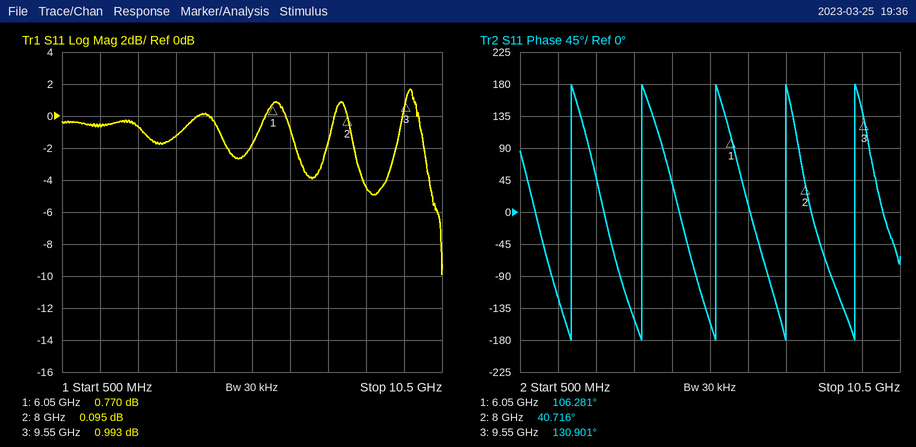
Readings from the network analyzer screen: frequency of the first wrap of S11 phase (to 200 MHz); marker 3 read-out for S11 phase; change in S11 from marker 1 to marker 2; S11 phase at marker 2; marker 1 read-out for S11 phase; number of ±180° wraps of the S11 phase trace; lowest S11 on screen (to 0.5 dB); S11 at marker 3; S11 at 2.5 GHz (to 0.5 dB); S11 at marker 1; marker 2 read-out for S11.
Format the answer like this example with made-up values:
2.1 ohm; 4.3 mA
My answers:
1.8 GHz; 130.901°; -0.675 dB; 40.716°; 106.281°; 5; -10.0 dB; 0.993 dB; -0.5 dB; 0.770 dB; 0.095 dB
